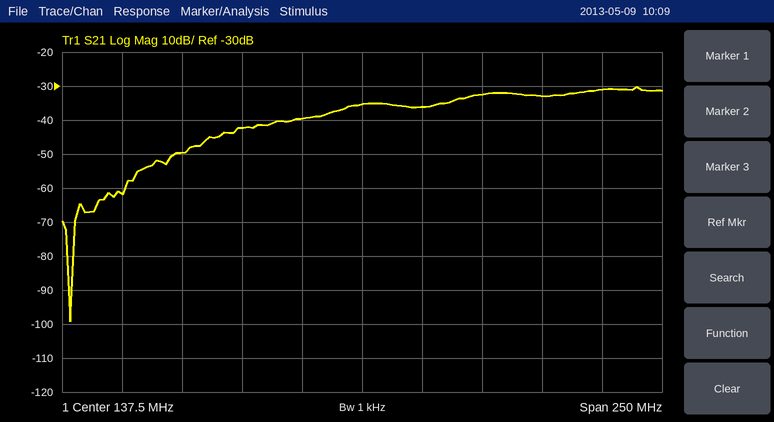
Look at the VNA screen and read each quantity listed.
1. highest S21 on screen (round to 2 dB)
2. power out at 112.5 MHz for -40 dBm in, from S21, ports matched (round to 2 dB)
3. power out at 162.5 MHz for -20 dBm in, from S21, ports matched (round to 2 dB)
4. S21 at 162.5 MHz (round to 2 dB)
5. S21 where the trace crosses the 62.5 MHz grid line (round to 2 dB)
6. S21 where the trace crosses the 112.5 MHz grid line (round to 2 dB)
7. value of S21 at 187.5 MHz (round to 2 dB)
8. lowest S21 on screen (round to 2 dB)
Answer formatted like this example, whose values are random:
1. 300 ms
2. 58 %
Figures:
1. -30 dB
2. -80 dBm
3. -56 dBm
4. -36 dB
5. -50 dB
6. -40 dB
7. -32 dB
8. -100 dB
